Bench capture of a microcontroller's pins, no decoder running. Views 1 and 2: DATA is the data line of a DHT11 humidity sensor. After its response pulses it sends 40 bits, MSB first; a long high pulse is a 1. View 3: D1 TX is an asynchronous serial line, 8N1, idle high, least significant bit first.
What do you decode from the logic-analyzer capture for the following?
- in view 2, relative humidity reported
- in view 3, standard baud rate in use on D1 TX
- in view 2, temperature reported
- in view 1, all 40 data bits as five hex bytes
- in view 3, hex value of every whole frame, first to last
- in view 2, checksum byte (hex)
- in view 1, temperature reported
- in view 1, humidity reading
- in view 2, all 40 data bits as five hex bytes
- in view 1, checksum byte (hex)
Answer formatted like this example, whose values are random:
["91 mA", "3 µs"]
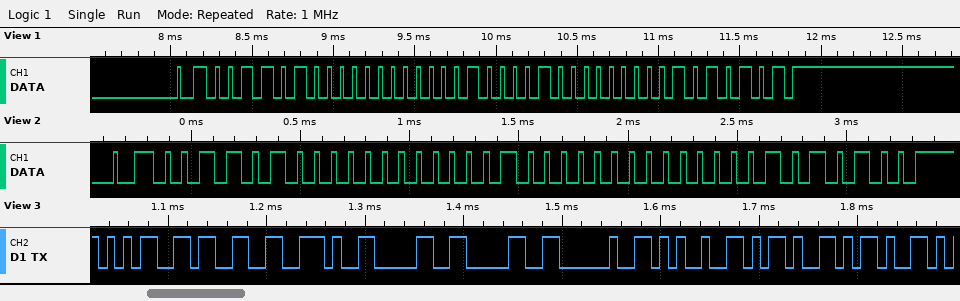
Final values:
["52 %", "115200 baud", "32.0 °C", "34 00 21 00 55", "35 33 2E 30 30 20 25 2D 2D", "0x54", "33.0 °C", "52 %", "34 00 20 00 54", "0x55"]
